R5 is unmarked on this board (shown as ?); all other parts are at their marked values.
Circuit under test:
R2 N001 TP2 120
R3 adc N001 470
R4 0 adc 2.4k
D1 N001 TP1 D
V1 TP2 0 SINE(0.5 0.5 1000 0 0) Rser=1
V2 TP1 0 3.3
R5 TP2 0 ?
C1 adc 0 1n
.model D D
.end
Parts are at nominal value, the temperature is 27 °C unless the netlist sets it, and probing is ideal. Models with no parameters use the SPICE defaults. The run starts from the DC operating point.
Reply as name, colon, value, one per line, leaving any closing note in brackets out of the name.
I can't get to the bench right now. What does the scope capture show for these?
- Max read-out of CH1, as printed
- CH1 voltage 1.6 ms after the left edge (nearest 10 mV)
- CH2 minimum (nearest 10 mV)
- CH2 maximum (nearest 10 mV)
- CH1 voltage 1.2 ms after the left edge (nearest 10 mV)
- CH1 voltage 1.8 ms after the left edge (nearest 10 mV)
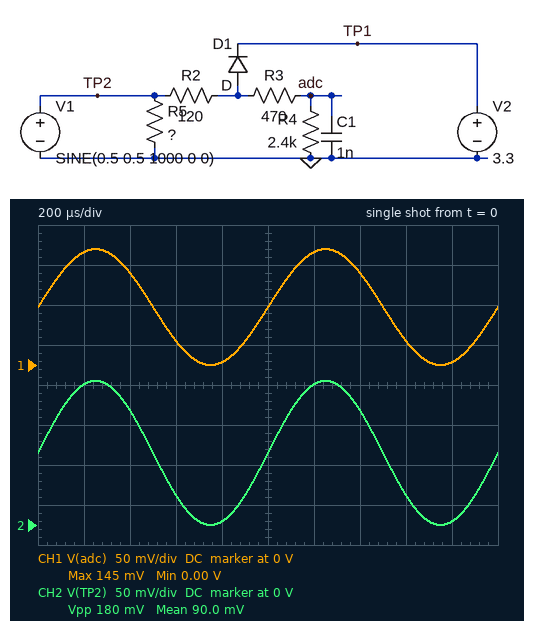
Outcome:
Max read-out of CH1, as printed: 145 mV
CH1 voltage 1.6 ms after the left edge: 30 mV
CH2 minimum: 0 V
CH2 maximum: 180 mV
CH1 voltage 1.2 ms after the left edge: 140 mV
CH1 voltage 1.8 ms after the left edge: 0 V
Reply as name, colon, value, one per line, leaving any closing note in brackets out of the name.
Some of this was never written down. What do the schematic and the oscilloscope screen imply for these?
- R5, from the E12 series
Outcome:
R5, from the E12 series: 0.22 Ω
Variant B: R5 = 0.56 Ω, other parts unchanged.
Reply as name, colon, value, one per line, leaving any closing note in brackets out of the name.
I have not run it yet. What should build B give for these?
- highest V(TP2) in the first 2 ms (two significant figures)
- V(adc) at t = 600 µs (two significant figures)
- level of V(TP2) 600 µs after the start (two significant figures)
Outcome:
highest V(TP2) in the first 2 ms: 360 mV
V(adc) at t = 600 µs: 60 mV
level of V(TP2) 600 µs after the start: 74 mV
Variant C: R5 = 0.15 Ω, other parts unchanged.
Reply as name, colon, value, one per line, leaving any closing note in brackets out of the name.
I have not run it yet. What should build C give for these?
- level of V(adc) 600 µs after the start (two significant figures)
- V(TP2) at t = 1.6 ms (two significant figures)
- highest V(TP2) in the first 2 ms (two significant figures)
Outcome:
level of V(adc) 600 µs after the start: 22 mV
V(TP2) at t = 1.6 ms: 27 mV
highest V(TP2) in the first 2 ms: 130 mV
